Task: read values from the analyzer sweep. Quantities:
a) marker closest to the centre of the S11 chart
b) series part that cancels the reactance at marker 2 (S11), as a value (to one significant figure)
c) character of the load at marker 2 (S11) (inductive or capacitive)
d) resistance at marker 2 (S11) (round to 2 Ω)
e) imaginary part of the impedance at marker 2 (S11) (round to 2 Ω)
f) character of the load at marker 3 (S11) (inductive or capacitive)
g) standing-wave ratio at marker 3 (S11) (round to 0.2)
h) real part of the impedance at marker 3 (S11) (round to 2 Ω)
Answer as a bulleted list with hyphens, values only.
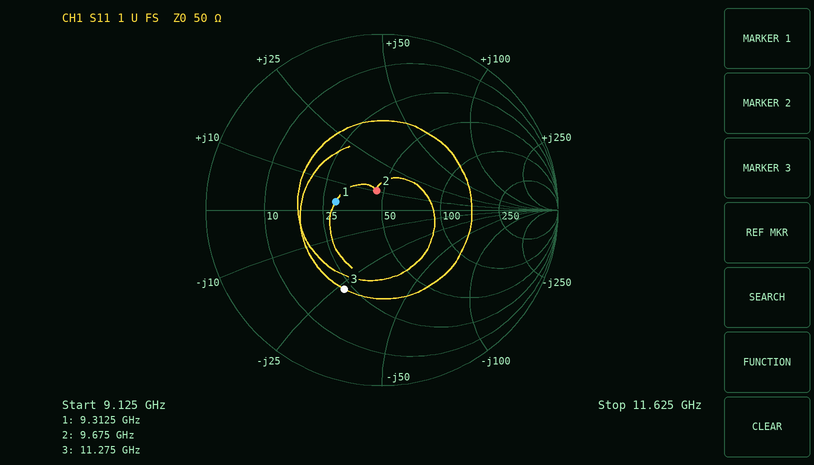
- marker 2
- 2 pF
- inductive
- 46 Ω
- +10 Ω
- capacitive
- 3.0
- 22 Ω
